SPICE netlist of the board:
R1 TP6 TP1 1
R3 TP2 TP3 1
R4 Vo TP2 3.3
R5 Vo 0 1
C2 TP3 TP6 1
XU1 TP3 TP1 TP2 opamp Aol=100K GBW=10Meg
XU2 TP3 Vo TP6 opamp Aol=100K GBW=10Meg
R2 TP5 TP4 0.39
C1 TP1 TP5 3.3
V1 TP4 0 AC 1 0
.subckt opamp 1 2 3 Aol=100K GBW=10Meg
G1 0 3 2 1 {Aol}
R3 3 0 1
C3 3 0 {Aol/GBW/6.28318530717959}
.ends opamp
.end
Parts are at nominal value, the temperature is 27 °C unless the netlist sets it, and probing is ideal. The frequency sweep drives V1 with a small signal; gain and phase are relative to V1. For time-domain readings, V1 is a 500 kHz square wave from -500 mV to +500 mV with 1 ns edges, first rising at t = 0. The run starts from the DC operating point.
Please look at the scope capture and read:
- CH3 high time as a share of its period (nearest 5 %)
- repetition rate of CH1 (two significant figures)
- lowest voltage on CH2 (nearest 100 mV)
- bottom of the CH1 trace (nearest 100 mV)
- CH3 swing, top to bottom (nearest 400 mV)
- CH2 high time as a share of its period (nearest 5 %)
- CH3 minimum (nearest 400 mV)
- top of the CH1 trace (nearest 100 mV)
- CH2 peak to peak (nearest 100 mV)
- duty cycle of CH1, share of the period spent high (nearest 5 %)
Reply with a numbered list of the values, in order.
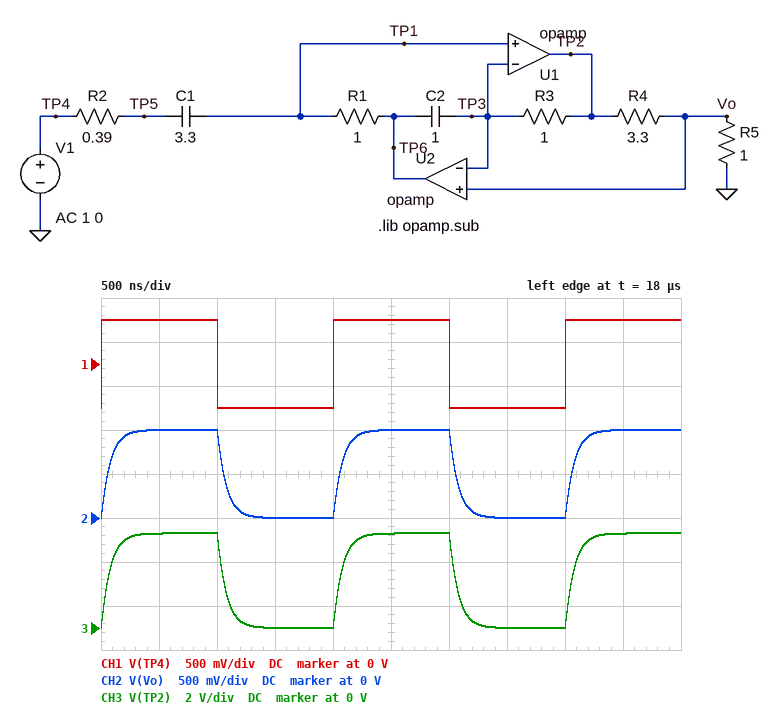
1. 50 %
2. 500 kHz
3. 0 V
4. -500 mV
5. 4.4 V
6. 50 %
7. 0 V
8. 500 mV
9. 1.0 V
10. 50 %
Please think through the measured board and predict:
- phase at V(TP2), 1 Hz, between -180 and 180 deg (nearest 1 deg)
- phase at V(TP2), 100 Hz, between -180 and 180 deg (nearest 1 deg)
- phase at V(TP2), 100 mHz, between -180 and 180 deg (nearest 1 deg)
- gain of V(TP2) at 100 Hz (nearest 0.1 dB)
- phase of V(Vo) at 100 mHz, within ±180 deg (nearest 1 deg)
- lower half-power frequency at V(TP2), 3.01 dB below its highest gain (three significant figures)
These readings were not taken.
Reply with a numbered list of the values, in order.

1. 12 deg
2. 0 deg
3. 127 deg
4. 12.7 dB
5. 127 deg
6. 148 mHz
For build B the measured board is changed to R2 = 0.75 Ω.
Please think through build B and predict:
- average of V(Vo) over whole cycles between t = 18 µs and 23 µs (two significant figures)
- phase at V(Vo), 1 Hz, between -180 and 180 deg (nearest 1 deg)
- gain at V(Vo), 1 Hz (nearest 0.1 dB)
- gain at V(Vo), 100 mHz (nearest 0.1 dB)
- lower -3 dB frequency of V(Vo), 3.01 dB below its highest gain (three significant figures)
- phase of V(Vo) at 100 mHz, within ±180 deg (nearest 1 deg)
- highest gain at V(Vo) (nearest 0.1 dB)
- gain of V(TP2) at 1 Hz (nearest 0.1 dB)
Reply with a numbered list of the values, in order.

1. 500 mV
2. 22 deg
3. -0.4 dB
4. -12.5 dB
5. 332 mHz
6. 111 deg
7. 0 dB
8. 12.2 dB
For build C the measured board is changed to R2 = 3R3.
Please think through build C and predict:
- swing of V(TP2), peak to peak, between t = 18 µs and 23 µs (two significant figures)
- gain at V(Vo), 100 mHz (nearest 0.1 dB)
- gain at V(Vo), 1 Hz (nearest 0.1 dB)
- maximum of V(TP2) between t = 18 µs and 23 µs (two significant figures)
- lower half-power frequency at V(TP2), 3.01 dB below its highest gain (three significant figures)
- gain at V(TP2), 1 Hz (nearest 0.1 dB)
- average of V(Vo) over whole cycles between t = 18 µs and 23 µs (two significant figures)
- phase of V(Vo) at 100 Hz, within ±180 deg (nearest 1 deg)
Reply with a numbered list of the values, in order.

1. 4.1 V
2. -24.8 dB
3. -6.0 dB
4. 4.2 V
5. 1.72 Hz
6. 6.7 dB
7. 500 mV
8. 1 deg
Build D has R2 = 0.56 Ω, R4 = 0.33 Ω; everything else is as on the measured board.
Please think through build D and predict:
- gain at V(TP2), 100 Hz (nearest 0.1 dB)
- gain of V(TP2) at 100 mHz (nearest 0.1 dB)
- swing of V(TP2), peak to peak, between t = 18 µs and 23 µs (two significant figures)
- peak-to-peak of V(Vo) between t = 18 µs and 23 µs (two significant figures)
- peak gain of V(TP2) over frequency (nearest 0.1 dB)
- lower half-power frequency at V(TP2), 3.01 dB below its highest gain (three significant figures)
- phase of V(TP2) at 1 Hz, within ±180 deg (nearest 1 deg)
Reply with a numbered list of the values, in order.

1. 2.5 dB
2. 4.4 dB
3. 1.5 V
4. 1.1 V
5. 7.5 dB
6. 42.7 mHz
7. 2 deg
